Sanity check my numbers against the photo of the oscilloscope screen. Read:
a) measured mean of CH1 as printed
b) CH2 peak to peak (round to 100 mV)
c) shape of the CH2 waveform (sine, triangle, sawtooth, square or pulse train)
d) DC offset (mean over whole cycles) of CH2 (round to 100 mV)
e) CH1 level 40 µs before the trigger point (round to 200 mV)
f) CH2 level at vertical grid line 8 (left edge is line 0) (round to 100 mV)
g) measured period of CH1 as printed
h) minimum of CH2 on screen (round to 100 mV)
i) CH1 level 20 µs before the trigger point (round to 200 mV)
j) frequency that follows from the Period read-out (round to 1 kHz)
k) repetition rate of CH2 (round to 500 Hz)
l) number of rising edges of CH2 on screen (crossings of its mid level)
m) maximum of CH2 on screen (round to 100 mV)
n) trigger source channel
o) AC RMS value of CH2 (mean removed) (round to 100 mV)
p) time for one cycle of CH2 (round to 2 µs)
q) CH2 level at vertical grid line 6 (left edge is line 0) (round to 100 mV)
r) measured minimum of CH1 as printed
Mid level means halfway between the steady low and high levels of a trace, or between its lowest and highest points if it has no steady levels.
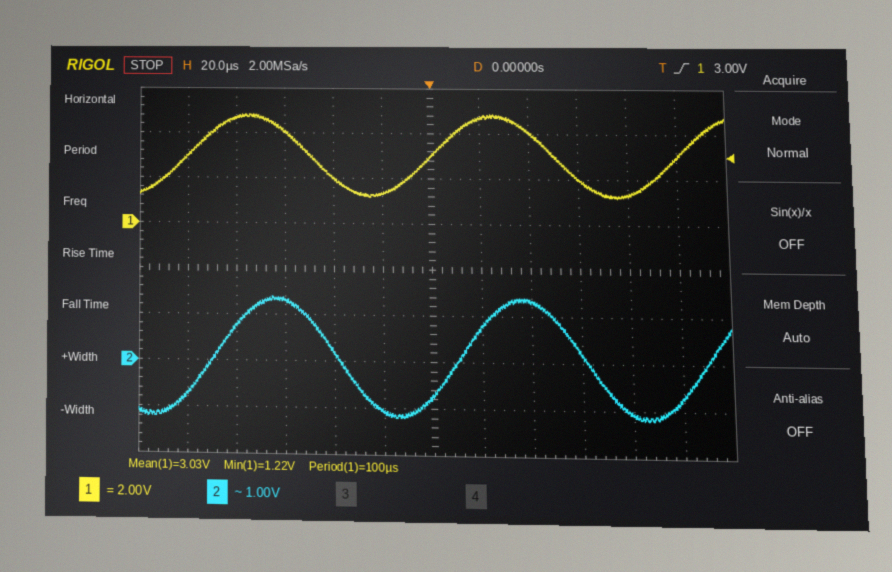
3.03 V
2.6 V
sine
100 mV
2.0 V
1.3 V
100 µs
-1.2 V
1.4 V
10 kHz
10.0 kHz
3
1.4 V
CH1
900 mV
100 µs
-700 mV
1.22 V
